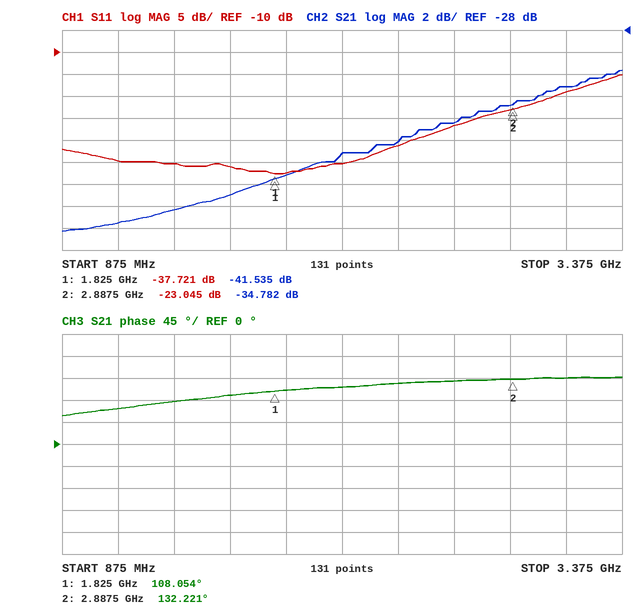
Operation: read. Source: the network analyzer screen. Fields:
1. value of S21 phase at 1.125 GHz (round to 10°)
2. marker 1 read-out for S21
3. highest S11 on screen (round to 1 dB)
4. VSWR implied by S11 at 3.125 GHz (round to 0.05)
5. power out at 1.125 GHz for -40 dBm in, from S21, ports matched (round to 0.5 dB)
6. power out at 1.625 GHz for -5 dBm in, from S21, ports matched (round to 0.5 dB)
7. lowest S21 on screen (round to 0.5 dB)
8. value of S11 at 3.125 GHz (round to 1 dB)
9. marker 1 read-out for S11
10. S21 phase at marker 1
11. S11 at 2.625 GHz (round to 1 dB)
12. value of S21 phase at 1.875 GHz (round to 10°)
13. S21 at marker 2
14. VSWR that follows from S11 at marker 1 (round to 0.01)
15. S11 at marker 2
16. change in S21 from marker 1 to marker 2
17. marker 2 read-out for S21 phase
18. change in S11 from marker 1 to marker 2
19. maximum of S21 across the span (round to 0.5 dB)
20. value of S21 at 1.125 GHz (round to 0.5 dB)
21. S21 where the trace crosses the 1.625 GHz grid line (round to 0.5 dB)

70°
-41.535 dB
-15 dB
1.25
-85.5 dBm
-48.0 dBm
-46.5 dB
-19 dB
-37.721 dB
108.054°
-27 dB
110°
-34.782 dB
1.03
-23.045 dB
6.753 dB
132.221°
14.676 dB
-31.5 dB
-45.5 dB
-43.0 dB
